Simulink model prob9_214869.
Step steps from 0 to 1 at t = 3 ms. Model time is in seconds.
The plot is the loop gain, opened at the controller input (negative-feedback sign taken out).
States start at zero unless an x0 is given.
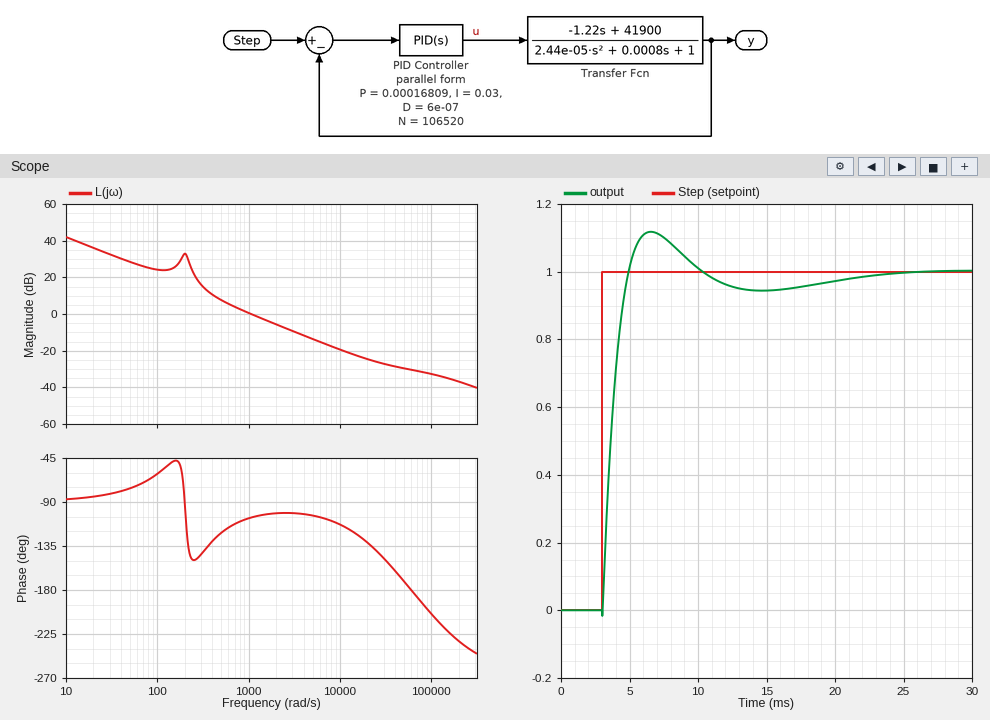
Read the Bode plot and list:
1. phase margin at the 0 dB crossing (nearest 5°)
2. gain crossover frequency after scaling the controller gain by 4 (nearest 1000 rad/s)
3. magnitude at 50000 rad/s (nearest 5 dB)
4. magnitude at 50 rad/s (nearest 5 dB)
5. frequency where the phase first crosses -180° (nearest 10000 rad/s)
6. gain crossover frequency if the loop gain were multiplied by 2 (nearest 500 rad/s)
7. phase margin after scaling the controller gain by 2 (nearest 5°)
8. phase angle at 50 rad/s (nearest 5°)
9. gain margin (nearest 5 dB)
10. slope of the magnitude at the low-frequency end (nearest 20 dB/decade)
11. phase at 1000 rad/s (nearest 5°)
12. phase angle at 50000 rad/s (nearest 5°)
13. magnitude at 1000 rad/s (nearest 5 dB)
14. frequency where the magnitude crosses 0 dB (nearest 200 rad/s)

75°
4000 rad/s
-30 dB
30 dB
60000 rad/s
2000 rad/s
80°
-75°
30 dB
-20 dB/decade
-105°
-170°
0 dB
1000 rad/s
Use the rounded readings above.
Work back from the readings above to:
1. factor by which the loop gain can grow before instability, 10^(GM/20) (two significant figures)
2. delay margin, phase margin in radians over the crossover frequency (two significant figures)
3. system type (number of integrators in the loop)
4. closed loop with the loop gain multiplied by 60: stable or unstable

32
0.0013 s
1
unstable
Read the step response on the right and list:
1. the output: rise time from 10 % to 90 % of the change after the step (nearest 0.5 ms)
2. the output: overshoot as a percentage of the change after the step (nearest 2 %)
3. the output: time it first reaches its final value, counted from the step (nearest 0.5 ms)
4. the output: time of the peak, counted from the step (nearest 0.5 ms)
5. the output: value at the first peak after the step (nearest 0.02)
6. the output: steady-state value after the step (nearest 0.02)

1.5 ms
12 %
2.0 ms
3.5 ms
1.12
1.00
